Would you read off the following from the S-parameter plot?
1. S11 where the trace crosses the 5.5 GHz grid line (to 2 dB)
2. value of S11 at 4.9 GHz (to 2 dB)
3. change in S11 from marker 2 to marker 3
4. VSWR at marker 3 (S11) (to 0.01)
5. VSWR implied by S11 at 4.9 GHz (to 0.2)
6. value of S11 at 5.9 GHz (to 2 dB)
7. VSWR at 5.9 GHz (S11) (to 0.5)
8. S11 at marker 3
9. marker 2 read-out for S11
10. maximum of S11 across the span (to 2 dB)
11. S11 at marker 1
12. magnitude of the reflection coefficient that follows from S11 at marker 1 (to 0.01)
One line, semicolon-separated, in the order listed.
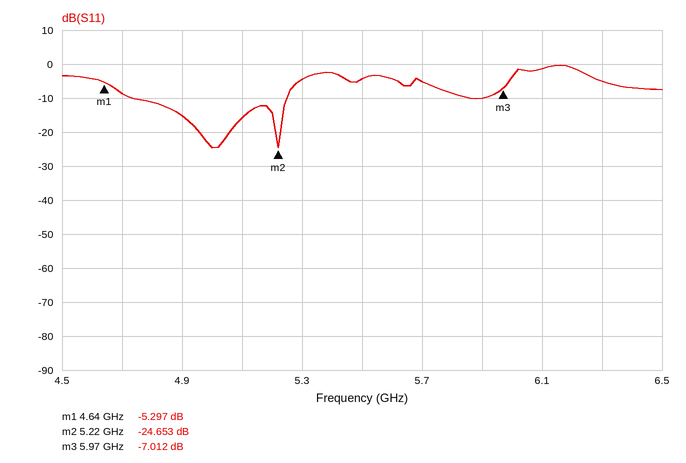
-4 dB; -16 dB; 17.641 dB; 2.61; 1.4; -10 dB; 2.0; -7.012 dB; -24.653 dB; 0 dB; -5.297 dB; 0.54
